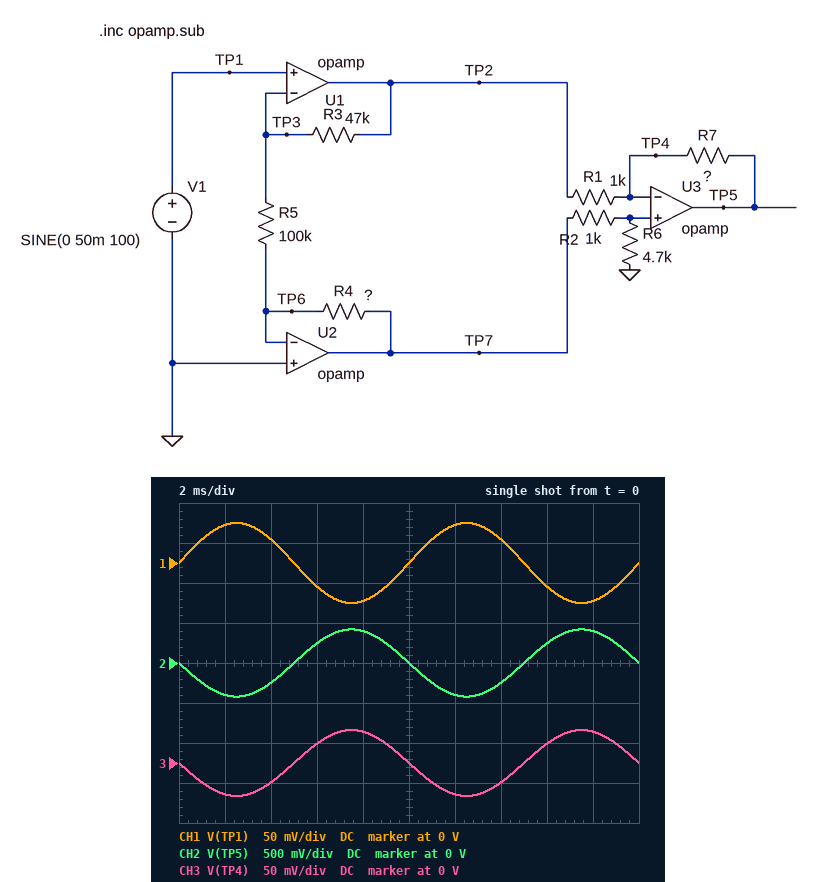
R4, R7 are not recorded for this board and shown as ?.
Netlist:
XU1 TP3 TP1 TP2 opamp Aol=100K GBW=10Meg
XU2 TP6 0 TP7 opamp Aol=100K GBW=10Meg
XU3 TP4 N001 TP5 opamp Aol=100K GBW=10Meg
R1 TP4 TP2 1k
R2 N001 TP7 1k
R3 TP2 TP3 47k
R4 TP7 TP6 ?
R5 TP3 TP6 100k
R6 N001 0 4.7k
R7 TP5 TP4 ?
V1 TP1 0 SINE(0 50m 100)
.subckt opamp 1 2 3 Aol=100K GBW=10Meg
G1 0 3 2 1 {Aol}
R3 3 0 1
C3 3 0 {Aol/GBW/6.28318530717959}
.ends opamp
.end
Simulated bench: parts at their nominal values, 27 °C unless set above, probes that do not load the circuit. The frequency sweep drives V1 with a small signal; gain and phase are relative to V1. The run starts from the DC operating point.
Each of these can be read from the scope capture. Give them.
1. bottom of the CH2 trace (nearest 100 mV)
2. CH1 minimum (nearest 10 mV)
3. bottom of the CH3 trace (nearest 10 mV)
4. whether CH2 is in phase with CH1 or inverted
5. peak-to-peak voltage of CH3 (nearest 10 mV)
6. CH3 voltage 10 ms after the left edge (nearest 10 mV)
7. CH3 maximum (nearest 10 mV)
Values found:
-400 mV
-50 mV
-40 mV
inverted
80 mV
0 V
40 mV
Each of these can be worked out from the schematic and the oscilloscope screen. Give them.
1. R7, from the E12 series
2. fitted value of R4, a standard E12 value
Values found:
3.3 kΩ
100 kΩ
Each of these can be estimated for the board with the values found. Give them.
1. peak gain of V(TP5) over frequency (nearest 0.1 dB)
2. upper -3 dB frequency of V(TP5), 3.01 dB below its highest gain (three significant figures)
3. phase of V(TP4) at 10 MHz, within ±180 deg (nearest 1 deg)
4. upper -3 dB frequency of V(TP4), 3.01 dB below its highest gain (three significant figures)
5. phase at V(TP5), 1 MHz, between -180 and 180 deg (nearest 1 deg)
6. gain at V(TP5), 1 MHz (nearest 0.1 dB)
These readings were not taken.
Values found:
18.5 dB
1.87 MHz
-38 deg
7.81 MHz
143 deg
17.5 dB
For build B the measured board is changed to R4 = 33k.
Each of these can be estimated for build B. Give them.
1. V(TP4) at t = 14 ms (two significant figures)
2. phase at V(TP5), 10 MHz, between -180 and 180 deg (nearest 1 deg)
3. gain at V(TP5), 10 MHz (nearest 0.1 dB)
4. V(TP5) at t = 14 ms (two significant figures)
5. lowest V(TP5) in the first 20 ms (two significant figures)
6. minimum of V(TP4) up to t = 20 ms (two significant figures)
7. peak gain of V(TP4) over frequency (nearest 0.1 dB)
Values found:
-8.0 mV
42 deg
-3.6 dB
-180 mV
-300 mV
-14 mV
-1.2 dB
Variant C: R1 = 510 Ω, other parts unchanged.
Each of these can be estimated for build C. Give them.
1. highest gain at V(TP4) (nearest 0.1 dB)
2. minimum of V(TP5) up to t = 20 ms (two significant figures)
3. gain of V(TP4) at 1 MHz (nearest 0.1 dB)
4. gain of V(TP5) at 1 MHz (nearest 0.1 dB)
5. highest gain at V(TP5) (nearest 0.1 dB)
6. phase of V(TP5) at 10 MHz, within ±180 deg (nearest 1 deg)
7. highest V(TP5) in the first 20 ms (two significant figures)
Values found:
1.4 dB
-780 mV
0.5 dB
21.7 dB
23.9 dB
30 deg
780 mV
